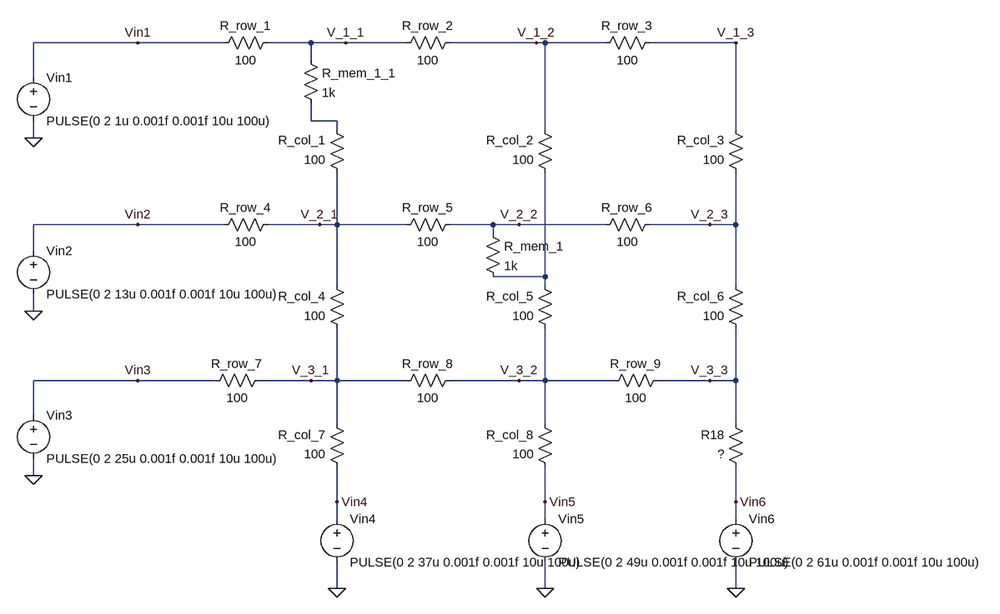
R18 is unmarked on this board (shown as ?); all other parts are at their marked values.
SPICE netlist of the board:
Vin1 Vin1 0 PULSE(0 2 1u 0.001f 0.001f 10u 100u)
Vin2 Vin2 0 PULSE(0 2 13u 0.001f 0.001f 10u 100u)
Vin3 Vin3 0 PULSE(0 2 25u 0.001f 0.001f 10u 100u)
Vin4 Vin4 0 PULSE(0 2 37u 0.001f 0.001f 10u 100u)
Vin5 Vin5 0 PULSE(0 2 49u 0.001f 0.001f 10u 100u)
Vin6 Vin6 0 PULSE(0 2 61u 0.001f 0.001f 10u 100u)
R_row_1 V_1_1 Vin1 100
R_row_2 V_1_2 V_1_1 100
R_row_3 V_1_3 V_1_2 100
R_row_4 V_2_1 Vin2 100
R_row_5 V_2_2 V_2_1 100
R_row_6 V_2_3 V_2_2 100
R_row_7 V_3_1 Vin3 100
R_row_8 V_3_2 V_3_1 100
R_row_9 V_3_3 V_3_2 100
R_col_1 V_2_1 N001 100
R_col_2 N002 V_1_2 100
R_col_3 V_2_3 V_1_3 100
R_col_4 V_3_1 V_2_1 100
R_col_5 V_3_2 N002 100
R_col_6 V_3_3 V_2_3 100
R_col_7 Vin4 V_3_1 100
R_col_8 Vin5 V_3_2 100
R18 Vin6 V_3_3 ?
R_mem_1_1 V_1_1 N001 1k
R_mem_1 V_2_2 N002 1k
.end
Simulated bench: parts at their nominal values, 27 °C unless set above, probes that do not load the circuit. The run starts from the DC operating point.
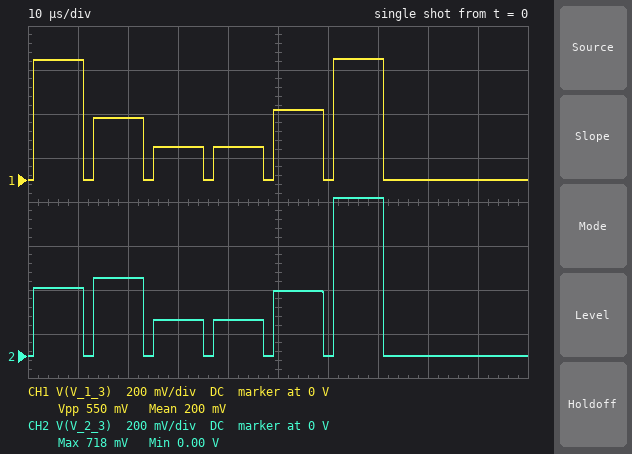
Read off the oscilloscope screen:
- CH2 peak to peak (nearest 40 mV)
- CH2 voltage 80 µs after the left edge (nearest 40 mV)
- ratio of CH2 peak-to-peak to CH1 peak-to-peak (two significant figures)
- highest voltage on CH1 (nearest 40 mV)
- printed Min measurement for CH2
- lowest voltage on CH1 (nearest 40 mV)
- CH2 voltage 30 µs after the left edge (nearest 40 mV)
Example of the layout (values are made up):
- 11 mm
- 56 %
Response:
- 720 mV
- 0 V
- 1.3
- 560 mV
- 0.00 V
- 0 V
- 160 mV
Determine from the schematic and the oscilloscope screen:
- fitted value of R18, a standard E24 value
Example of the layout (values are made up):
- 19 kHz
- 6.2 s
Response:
- 75 Ω
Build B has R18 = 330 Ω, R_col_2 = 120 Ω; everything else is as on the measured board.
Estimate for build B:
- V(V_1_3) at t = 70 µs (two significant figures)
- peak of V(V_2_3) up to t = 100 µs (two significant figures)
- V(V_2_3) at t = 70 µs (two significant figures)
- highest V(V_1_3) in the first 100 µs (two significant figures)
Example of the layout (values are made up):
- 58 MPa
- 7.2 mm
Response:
- 220 mV
- 450 mV
- 290 mV
- 610 mV
